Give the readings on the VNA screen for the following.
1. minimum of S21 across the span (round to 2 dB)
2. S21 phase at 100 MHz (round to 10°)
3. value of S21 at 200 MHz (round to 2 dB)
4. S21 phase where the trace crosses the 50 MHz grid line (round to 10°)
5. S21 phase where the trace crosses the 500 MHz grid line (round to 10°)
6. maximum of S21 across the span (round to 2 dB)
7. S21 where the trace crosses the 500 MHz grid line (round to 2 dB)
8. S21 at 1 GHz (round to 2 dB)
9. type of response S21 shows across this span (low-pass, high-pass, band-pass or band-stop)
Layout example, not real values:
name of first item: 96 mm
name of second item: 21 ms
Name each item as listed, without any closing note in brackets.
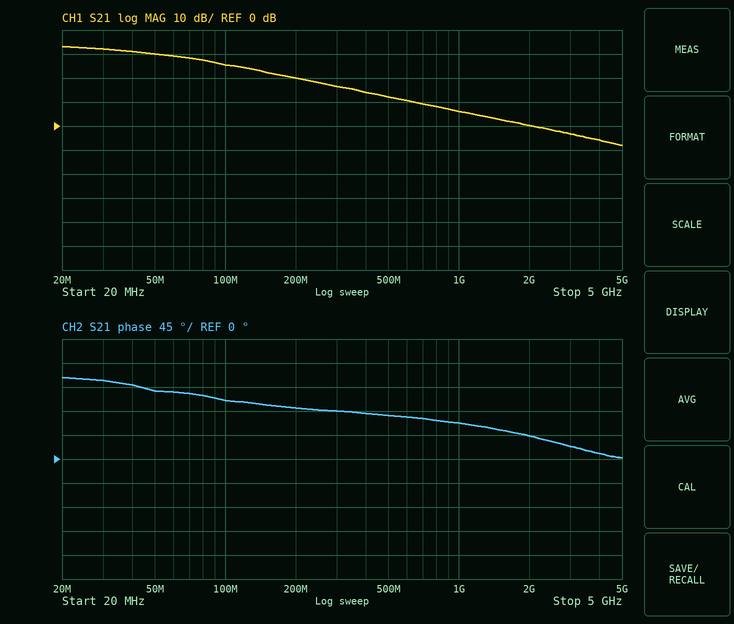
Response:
minimum of S21 across the span: -8 dB
S21 phase at 100 MHz: 110°
value of S21 at 200 MHz: 20 dB
S21 phase where the trace crosses the 50 MHz grid line: 130°
S21 phase where the trace crosses the 500 MHz grid line: 80°
maximum of S21 across the span: 34 dB
S21 where the trace crosses the 500 MHz grid line: 12 dB
S21 at 1 GHz: 6 dB
type of response S21 shows across this span: low-pass
